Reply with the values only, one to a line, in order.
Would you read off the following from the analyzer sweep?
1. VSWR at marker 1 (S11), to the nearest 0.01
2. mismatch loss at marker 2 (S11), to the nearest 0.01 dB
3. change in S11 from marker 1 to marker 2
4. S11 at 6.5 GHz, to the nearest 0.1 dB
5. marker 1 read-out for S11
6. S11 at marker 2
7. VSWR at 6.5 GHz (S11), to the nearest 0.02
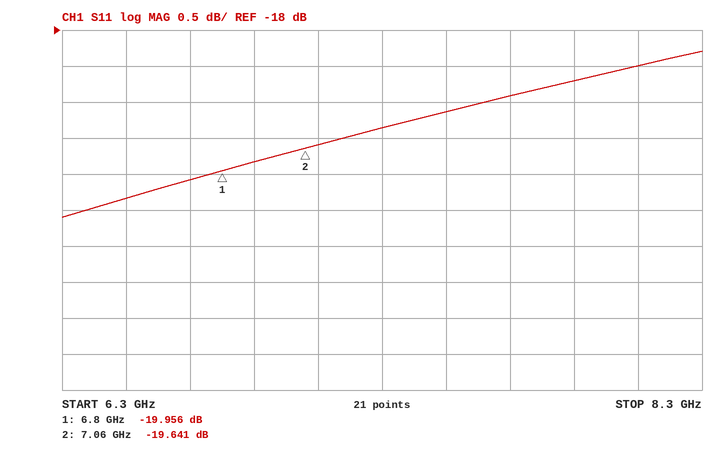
1.22
0.05 dB
0.315 dB
-20.3 dB
-19.956 dB
-19.641 dB
1.22
